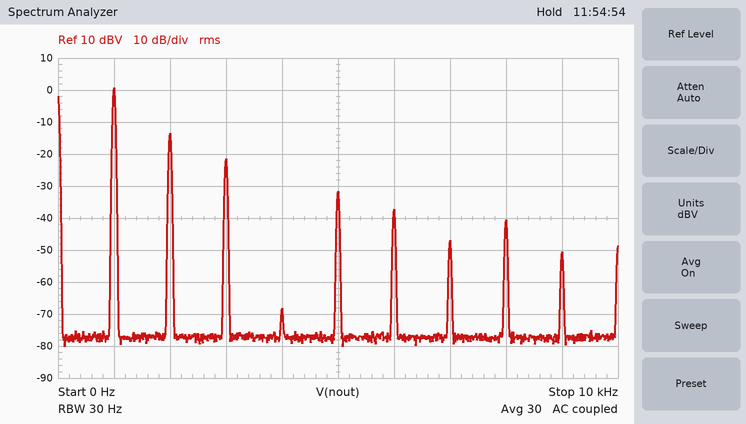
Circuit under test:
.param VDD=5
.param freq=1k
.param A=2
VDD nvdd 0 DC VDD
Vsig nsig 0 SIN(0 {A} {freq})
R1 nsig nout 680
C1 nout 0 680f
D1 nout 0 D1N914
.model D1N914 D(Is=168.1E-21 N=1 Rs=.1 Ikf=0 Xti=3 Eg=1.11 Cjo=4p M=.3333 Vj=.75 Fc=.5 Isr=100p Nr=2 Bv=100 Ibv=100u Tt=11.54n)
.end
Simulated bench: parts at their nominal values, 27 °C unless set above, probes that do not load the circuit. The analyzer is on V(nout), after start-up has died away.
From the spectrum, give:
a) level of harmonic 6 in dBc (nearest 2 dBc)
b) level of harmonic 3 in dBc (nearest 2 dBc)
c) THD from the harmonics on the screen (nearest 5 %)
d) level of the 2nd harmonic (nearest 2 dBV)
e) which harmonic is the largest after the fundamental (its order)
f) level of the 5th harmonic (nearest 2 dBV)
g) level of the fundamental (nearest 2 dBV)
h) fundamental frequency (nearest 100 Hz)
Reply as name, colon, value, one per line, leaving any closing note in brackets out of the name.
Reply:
level of harmonic 6 in dBc: -38 dBc
level of harmonic 3 in dBc: -22 dBc
THD from the harmonics on the screen: 20 %
level of the 2nd harmonic: -14 dBV
which harmonic is the largest after the fundamental: 2
level of the 5th harmonic: -32 dBV
level of the fundamental: 0 dBV
fundamental frequency: 1.0 kHz
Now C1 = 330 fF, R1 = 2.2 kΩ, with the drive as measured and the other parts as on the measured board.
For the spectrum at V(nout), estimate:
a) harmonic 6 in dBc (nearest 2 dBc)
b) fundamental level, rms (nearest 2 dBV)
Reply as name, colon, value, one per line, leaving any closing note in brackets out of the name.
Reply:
harmonic 6 in dBc: -40 dBc
fundamental level, rms: 0 dBV
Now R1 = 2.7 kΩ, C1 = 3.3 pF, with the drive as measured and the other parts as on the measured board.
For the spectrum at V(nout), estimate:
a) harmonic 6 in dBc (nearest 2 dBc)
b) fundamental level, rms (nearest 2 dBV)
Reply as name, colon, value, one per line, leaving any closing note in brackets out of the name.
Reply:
harmonic 6 in dBc: -40 dBc
fundamental level, rms: 0 dBV
